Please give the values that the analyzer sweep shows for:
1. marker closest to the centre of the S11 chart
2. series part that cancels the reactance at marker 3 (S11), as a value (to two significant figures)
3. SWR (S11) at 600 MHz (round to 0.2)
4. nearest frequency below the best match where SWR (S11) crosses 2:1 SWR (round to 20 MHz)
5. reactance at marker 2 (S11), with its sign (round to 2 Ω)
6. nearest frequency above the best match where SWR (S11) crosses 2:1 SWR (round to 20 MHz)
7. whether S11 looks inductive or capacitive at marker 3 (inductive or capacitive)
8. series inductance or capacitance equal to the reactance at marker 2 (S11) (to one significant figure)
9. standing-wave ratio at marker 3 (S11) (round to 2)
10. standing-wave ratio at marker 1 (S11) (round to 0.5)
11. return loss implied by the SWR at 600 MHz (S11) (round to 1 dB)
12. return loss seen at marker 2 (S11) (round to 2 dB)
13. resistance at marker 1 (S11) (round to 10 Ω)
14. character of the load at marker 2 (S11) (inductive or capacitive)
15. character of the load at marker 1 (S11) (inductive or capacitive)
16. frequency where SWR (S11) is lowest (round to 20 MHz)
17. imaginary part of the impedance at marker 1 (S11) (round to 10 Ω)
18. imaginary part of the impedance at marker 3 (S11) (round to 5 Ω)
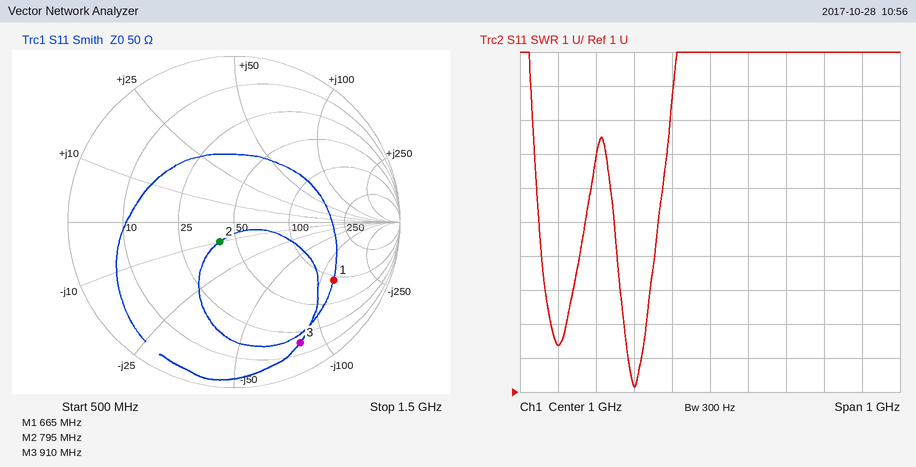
marker 2
14 nH
2.4
780 MHz
-10 Ω
820 MHz
capacitive
20 pF
10
5.5
8 dB
16 dB
90 Ω
capacitive
capacitive
800 MHz
-120 Ω
-80 Ω
